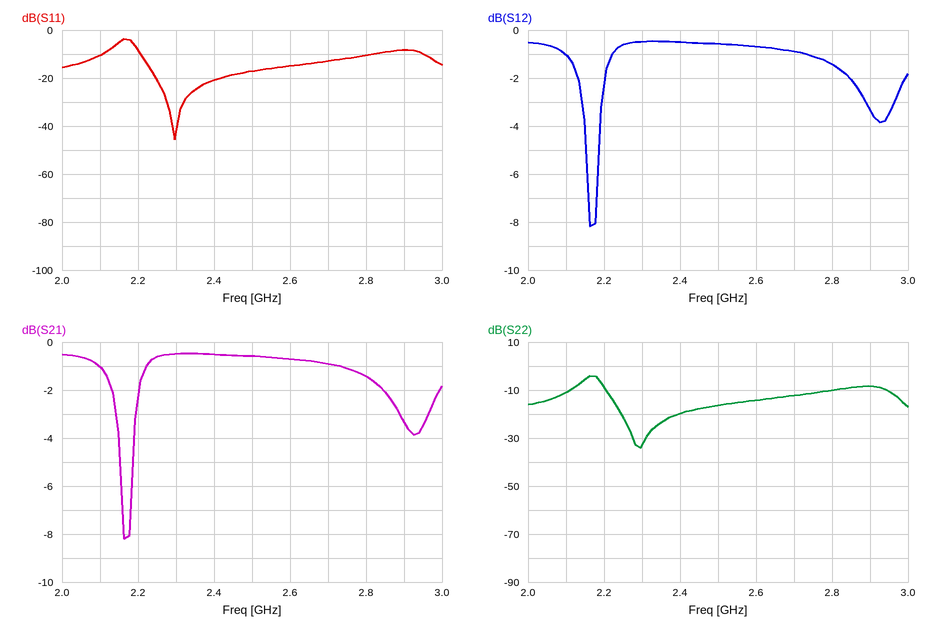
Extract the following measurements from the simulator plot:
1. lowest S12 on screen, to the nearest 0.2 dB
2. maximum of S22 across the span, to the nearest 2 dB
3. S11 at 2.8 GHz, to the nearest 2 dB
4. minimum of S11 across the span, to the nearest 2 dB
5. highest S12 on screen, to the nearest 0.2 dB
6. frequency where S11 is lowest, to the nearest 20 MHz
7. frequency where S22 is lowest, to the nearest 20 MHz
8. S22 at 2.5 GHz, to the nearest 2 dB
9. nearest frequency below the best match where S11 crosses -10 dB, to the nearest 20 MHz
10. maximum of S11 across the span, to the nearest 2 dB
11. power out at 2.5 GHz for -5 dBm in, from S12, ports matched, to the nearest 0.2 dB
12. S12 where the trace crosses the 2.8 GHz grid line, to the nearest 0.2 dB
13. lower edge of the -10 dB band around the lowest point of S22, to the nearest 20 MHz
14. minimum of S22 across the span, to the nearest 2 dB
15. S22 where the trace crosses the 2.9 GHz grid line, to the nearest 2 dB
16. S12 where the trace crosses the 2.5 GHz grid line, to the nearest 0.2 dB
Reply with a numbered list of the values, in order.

1. -8.2 dB
2. -4 dB
3. -10 dB
4. -46 dB
5. -0.4 dB
6. 2.30 GHz
7. 2.30 GHz
8. -16 dB
9. 2.20 GHz
10. -4 dB
11. -5.6 dBm
12. -1.4 dB
13. 2.20 GHz
14. -34 dB
15. -8 dB
16. -0.6 dB
